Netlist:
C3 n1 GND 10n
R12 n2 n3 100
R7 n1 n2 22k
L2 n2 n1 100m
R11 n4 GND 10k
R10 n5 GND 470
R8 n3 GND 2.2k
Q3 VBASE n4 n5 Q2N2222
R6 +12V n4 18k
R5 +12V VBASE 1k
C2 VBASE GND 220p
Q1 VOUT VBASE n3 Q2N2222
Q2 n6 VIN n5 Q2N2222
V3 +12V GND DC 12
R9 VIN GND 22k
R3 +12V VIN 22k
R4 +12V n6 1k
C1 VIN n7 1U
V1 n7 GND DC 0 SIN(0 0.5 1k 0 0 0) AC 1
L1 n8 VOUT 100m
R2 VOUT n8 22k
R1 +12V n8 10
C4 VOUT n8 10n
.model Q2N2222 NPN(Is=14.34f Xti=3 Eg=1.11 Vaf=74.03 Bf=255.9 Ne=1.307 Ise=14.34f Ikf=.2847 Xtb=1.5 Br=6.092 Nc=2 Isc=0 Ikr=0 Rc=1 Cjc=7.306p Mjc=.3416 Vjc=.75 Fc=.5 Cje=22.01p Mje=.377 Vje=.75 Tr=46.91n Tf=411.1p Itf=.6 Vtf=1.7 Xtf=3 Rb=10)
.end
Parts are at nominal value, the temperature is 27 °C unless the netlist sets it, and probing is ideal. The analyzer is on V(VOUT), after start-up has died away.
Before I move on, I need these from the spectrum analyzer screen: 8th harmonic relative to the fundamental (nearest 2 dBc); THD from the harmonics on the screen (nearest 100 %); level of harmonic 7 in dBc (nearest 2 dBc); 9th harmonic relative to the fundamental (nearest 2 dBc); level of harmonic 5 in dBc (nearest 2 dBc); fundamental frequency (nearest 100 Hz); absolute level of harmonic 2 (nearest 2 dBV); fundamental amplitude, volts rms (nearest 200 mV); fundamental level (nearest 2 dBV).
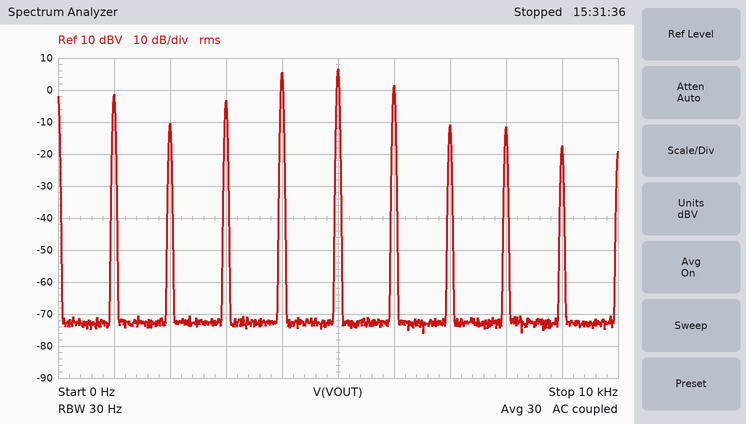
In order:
-10 dBc
400 %
-10 dBc
-16 dBc
8 dBc
1.0 kHz
-10 dBV
800 mV
-2 dBV
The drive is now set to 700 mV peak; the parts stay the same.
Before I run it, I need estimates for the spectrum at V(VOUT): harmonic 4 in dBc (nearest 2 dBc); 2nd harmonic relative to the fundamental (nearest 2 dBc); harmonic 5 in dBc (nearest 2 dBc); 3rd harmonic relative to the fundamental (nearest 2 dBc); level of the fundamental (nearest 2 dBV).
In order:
8 dBc
0 dBc
12 dBc
-6 dBc
-2 dBV
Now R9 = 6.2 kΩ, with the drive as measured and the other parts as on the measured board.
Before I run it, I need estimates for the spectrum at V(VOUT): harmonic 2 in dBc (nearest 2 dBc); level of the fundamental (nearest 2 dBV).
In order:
-16 dBc
-100 dBV
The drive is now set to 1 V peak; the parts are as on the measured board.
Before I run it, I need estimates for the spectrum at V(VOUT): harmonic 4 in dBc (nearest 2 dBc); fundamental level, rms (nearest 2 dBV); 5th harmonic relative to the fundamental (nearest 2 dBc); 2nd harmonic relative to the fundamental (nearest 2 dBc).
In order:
12 dBc
-2 dBV
12 dBc
-4 dBc
